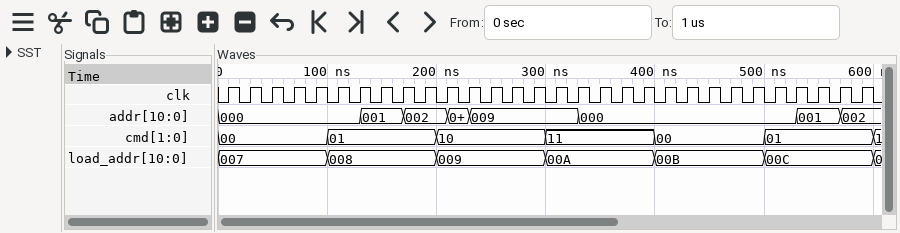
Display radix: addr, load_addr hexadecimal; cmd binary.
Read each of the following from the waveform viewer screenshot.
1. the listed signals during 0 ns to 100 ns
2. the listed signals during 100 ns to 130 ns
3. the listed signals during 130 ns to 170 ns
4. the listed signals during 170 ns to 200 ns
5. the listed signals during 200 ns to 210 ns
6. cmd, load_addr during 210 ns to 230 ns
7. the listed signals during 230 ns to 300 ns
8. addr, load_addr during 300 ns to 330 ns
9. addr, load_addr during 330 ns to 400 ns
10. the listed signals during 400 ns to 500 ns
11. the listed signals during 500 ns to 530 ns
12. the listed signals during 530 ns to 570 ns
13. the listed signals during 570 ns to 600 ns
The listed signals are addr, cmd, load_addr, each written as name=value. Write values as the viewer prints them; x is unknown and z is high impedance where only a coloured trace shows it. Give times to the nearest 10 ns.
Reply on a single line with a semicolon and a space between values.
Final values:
addr=000, cmd=00, load_addr=007; addr=000, cmd=01, load_addr=008; addr=001, cmd=01, load_addr=008; addr=002, cmd=01, load_addr=008; addr=002, cmd=10, load_addr=009; cmd=10, load_addr=009; addr=009, cmd=10, load_addr=009; addr=009, load_addr=00A; addr=000, load_addr=00A; addr=000, cmd=00, load_addr=00B; addr=000, cmd=01, load_addr=00C; addr=001, cmd=01, load_addr=00C; addr=002, cmd=01, load_addr=00C
